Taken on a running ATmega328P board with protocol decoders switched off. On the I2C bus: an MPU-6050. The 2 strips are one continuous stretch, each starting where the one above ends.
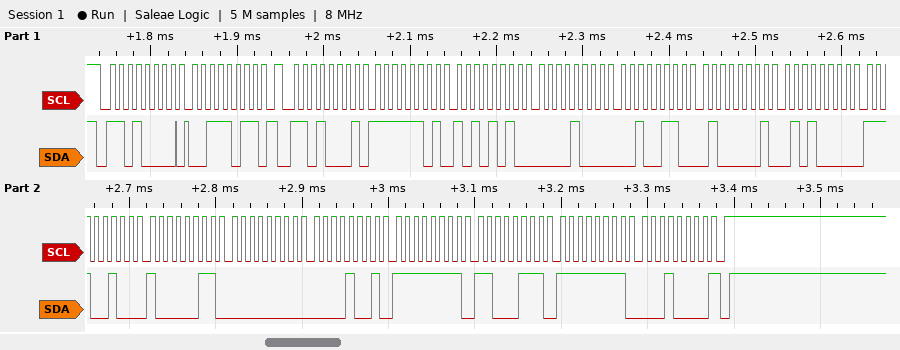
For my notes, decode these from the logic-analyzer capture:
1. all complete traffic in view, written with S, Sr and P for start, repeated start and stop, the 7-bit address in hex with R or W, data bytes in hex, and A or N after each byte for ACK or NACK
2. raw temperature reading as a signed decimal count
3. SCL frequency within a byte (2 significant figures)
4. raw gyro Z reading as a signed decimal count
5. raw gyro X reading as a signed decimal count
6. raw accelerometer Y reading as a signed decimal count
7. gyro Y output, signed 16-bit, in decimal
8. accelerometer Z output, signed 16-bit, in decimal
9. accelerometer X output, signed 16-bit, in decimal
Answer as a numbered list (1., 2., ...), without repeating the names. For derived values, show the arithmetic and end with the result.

1. S 68W A 3B A Sr 68R A FD A AA A 08 A 26 A 41 A 50 A E4 A 83 A 00 A 09 A FF A C7 A FF A 10 N P
2. 0xE483 = -7037
3. 100 kHz
4. 0xFF10 = -240
5. 0x0009 = 9
6. 0x0826 = 2086
7. 0xFFC7 = -57
8. 0x4150 = 16720
9. 0xFDAA = -598
